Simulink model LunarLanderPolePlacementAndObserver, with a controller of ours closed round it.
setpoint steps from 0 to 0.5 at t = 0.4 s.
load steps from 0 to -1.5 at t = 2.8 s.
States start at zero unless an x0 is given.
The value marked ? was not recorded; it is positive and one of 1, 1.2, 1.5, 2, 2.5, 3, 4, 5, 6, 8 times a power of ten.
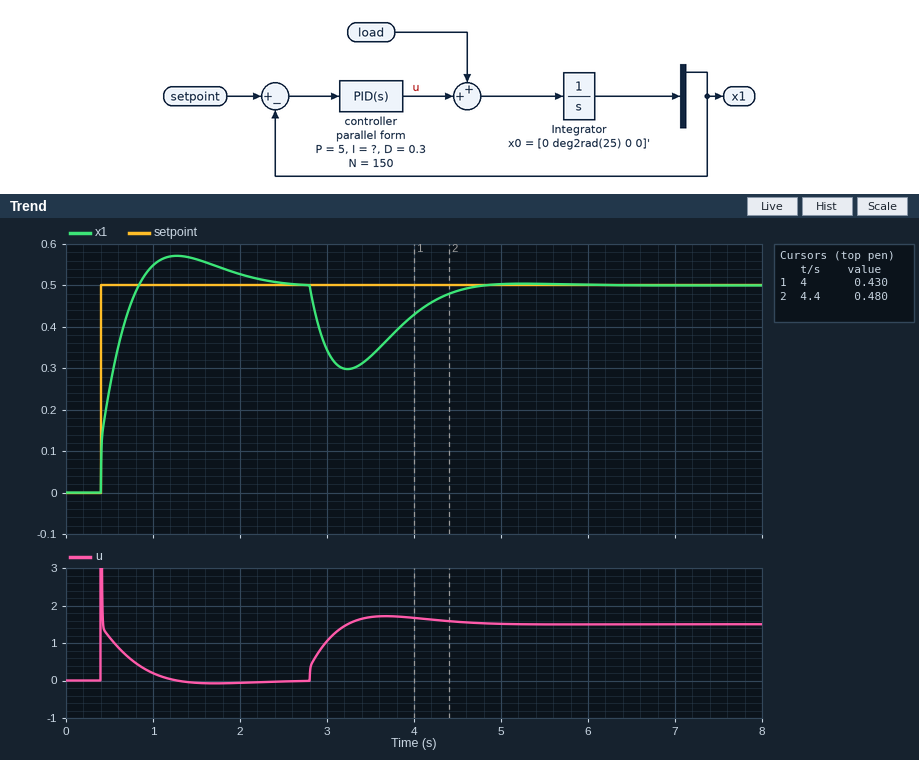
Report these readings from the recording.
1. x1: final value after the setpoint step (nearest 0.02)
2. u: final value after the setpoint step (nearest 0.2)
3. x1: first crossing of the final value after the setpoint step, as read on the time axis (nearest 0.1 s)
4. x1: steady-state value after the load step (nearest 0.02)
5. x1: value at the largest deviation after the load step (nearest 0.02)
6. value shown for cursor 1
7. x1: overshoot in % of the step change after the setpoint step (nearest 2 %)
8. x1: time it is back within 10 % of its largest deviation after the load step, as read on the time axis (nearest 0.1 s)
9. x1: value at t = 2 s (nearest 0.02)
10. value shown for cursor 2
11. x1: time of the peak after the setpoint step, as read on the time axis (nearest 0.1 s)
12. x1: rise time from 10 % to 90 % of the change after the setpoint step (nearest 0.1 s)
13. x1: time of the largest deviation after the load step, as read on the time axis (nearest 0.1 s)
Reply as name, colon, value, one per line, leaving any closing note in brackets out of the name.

x1: final value after the setpoint step: 0.50
u: final value after the setpoint step: 0.0
x1: first crossing of the final value after the setpoint step, as read on the time axis: 0.8 s
x1: steady-state value after the load step: 0.50
x1: value at the largest deviation after the load step: 0.30
value shown for cursor 1: 0.430
x1: overshoot in % of the step change after the setpoint step: 14 %
x1: time it is back within 10 % of its largest deviation after the load step, as read on the time axis: 4.4 s
x1: value at t = 2 s: 0.52
value shown for cursor 2: 0.480
x1: time of the peak after the setpoint step, as read on the time axis: 1.3 s
x1: rise time from 10 % to 90 % of the change after the setpoint step: 0.3 s
x1: time of the largest deviation after the load step, as read on the time axis: 3.2 s
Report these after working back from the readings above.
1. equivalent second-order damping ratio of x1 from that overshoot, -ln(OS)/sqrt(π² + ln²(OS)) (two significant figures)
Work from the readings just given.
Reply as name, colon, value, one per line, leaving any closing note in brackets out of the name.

equivalent second-order damping ratio of x1 from that overshoot, -ln(OS)/sqrt(π² + ln²(OS)): 0.53
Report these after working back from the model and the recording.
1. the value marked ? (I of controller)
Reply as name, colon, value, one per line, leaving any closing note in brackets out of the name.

the value marked ?: 8
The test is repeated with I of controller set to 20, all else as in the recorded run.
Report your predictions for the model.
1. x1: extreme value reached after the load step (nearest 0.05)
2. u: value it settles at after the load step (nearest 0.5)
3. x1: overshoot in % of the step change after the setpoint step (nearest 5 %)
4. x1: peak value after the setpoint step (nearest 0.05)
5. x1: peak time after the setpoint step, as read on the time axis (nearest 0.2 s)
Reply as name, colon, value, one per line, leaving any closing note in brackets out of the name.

x1: extreme value reached after the load step: 0.35
u: value it settles at after the load step: 1.5
x1: overshoot in % of the step change after the setpoint step: 25 %
x1: peak value after the setpoint step: 0.60
x1: peak time after the setpoint step, as read on the time axis: 1.0 s
